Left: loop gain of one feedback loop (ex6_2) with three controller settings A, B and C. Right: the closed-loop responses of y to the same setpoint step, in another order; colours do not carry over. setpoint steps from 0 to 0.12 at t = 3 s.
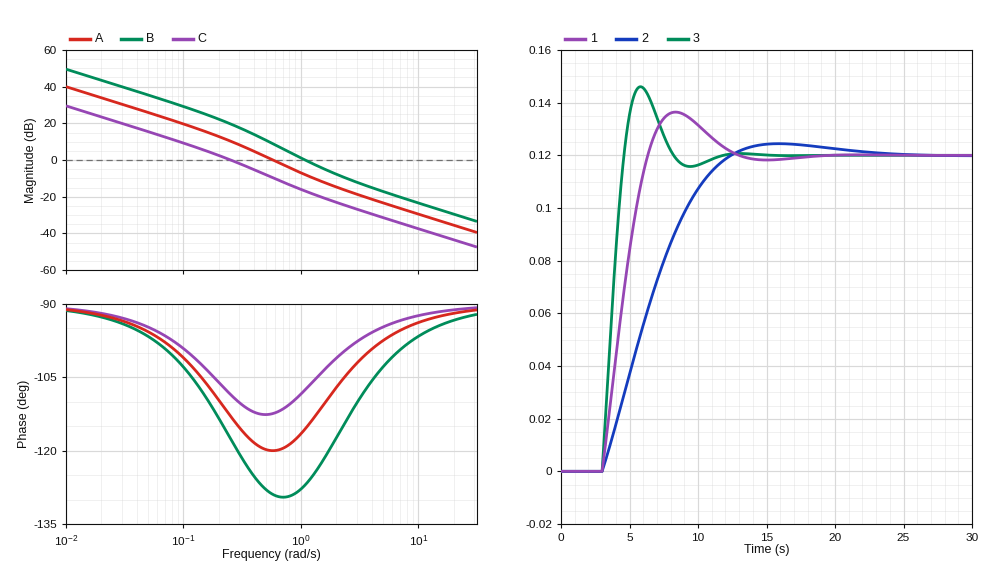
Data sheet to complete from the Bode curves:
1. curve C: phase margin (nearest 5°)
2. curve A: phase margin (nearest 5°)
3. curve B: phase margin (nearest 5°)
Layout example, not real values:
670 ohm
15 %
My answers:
70°
60°
55°
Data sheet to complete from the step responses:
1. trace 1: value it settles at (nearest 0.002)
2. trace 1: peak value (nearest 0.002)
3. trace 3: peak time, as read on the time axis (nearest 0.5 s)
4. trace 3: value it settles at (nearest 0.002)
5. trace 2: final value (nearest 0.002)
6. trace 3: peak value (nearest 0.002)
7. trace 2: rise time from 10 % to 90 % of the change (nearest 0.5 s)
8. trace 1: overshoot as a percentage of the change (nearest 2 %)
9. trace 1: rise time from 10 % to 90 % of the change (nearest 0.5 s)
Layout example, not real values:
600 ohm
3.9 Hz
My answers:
0.120
0.136
6.0 s
0.120
0.120
0.146
6.5 s
14 %
2.5 s
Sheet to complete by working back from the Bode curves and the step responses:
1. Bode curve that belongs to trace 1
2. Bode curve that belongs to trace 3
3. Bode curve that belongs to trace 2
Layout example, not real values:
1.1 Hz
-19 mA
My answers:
A
B
C
